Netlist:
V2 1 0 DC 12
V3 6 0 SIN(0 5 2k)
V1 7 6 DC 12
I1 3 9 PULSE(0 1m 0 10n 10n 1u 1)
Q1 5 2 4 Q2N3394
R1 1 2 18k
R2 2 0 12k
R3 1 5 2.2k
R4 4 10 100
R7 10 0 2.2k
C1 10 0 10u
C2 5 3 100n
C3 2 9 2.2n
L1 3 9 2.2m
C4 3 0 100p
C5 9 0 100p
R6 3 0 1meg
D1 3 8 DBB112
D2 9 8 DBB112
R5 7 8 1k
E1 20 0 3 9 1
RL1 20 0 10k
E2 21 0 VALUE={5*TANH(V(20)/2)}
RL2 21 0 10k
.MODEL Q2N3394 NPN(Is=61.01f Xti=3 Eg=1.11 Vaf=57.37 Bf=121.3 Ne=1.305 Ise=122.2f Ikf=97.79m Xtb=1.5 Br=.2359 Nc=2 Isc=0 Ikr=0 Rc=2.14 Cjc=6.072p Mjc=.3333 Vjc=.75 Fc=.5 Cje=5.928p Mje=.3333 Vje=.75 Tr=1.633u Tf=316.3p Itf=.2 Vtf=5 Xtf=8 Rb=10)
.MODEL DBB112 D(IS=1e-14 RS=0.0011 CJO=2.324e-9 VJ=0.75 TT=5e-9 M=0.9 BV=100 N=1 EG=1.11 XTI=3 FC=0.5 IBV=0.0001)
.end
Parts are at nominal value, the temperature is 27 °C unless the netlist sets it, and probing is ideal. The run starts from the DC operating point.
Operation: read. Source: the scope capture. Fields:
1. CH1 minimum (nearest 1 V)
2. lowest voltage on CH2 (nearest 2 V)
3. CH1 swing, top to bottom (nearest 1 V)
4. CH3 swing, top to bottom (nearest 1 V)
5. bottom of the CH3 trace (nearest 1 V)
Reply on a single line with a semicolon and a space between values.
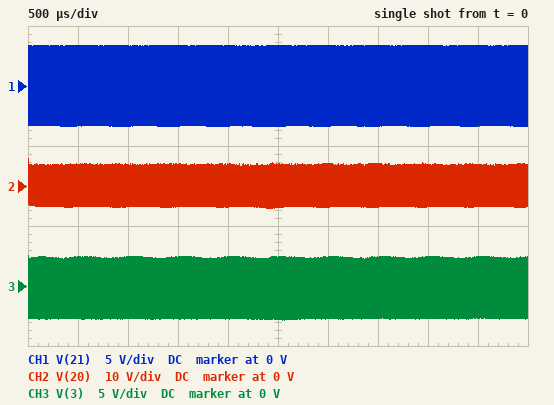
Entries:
-5 V; -6 V; 10 V; 8 V; -4 V
